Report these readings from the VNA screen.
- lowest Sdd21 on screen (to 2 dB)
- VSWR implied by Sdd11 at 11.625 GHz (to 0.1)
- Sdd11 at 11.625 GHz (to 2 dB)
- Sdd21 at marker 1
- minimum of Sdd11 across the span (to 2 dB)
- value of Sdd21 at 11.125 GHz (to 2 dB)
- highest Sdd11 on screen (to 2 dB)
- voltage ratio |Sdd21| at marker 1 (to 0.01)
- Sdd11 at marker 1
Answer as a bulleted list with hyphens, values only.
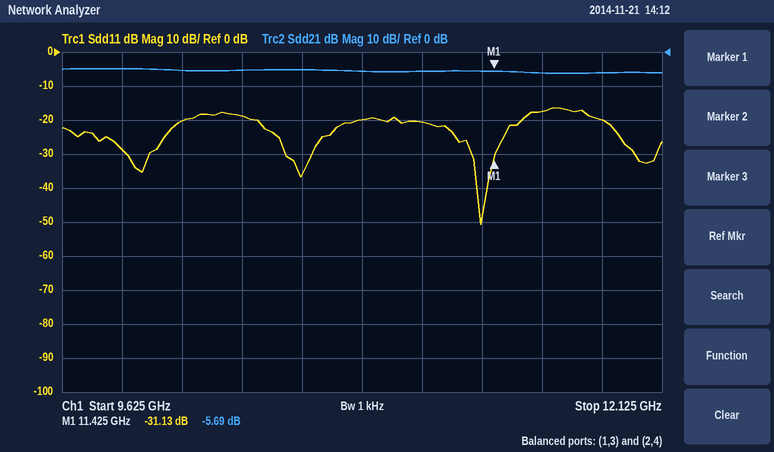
- -6 dB
- 1.3
- -18 dB
- -5.69 dB
- -50 dB
- -6 dB
- -16 dB
- 0.52
- -31.13 dB
